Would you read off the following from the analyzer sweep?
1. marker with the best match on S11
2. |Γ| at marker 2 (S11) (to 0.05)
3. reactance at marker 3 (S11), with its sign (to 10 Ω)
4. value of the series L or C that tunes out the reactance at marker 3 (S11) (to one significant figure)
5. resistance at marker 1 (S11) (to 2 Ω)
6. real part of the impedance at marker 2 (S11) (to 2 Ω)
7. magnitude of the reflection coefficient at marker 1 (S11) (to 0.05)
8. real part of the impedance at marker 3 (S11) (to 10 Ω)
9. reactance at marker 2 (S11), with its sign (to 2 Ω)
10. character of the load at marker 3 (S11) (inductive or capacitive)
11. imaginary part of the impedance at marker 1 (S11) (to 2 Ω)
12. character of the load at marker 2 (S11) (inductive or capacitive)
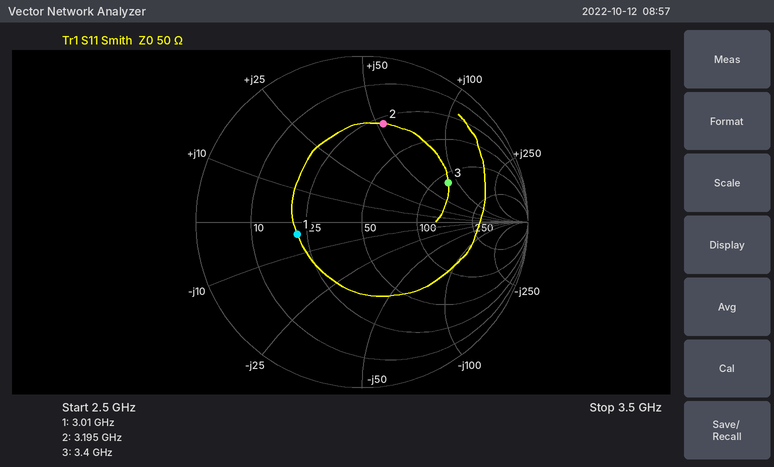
marker 1
0.60
+80 Ω
600 fF
22 Ω
28 Ω
0.40
120 Ω
+54 Ω
inductive
-4 Ω
inductive
